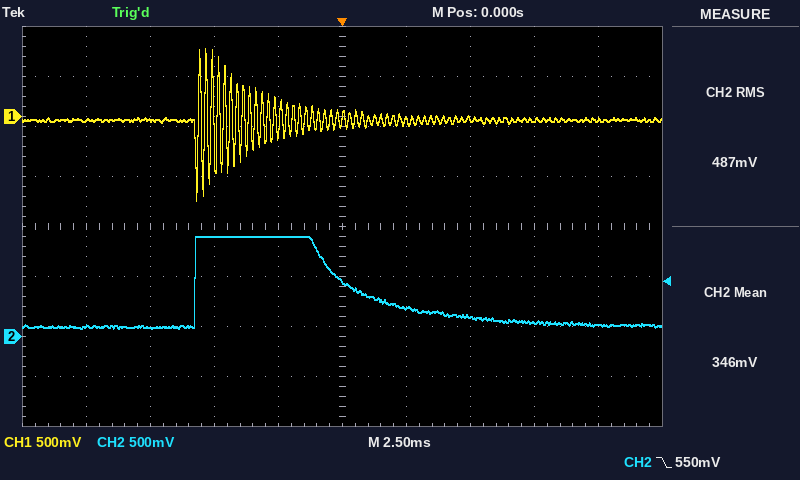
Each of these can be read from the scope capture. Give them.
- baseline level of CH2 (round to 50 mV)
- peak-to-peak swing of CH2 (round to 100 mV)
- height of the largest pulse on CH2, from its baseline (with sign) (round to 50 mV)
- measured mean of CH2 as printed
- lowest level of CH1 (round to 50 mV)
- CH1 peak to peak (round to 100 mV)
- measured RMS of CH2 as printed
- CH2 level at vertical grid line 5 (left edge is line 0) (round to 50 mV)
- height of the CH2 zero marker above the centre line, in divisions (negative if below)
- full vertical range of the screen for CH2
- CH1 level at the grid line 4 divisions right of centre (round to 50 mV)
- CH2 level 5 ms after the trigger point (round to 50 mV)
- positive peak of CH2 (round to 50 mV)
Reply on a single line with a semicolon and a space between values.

100 mV; 900 mV; +900 mV; 346 mV; -850 mV; 1.50 V; 487 mV; 550 mV; -2.2 div; 4 V; -50 mV; 200 mV; 1.00 V
